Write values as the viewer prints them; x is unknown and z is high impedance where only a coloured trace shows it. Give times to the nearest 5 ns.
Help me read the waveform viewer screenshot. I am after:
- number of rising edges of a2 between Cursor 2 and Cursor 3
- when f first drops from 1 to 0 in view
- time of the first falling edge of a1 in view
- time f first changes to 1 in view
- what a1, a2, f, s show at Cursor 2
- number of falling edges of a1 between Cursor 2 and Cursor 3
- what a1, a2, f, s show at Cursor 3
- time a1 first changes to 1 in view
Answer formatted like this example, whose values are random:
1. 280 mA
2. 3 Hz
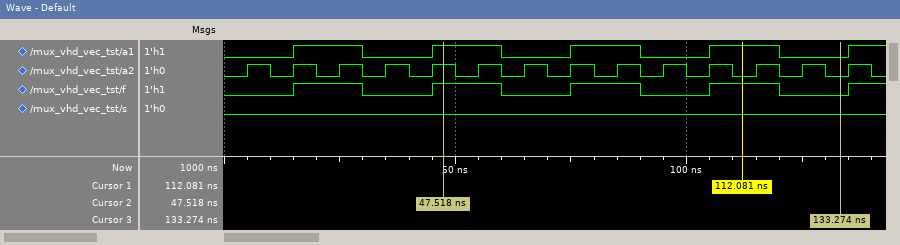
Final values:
1. 8
2. 30 ns
3. 30 ns
4. 15 ns
5. a1=1, a2=1, f=1, s=0
6. 3
7. a1=0, a2=0, f=0, s=0
8. 15 ns
